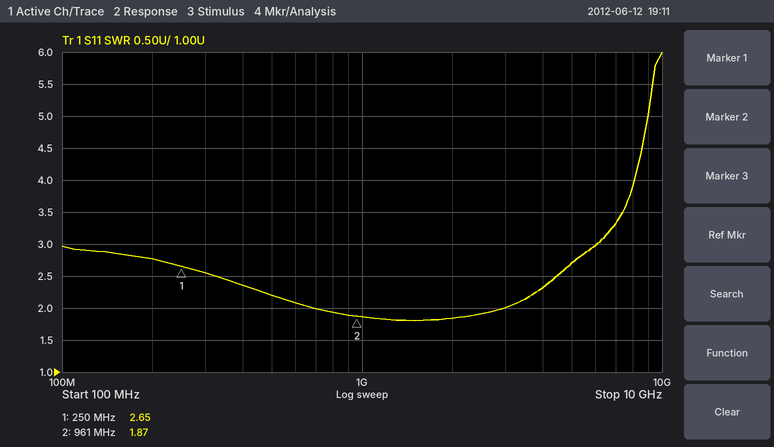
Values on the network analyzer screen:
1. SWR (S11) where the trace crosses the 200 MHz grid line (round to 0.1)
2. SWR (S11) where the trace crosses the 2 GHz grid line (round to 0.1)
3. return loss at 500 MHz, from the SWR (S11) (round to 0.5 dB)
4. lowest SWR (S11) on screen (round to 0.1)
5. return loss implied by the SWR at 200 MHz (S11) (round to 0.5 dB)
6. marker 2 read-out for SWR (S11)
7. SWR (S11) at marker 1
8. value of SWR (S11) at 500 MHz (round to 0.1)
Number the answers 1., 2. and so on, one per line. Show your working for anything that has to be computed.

1. 2.8
2. 1.8
3. −20 log10((2.2 − 1)/(2.2 + 1)) ≈ 8.5 dB
4. 1.8
5. −20 log10((2.8 − 1)/(2.8 + 1)) ≈ 6.5 dB
6. 1.87
7. 2.65
8. 2.2
